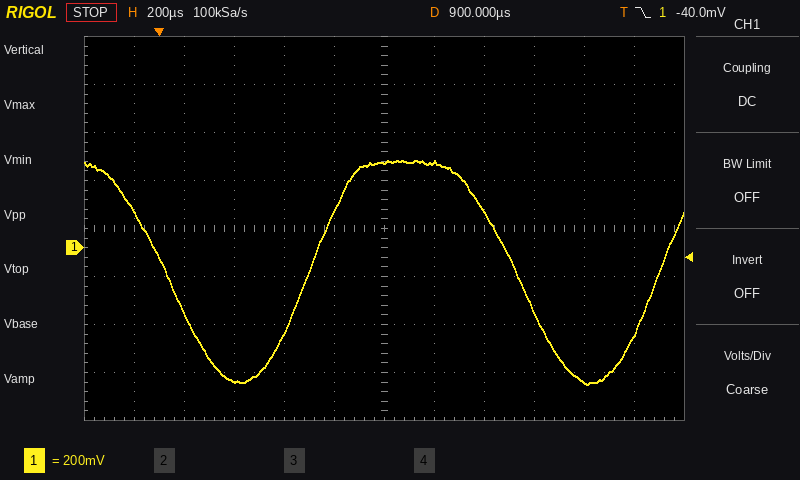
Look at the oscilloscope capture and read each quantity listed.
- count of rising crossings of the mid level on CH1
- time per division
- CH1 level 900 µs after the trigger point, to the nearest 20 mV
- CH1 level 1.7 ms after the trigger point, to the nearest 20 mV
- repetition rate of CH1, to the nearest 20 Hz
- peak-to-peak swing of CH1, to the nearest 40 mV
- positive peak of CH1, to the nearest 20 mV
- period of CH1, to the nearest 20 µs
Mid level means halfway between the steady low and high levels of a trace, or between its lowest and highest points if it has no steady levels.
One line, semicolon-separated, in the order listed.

2; 200 µs; 360 mV; -560 mV; 720 Hz; 920 mV; 360 mV; 1.40 ms
